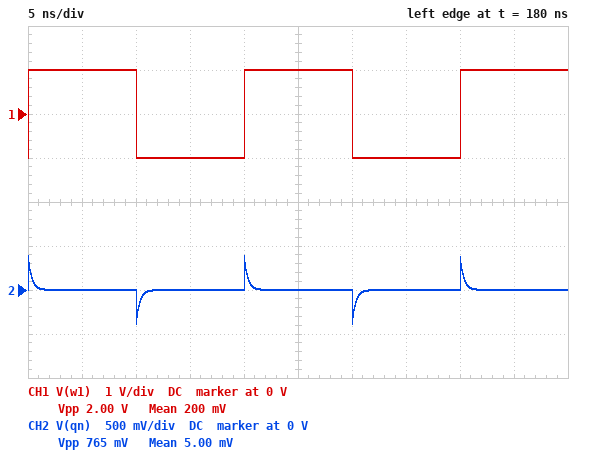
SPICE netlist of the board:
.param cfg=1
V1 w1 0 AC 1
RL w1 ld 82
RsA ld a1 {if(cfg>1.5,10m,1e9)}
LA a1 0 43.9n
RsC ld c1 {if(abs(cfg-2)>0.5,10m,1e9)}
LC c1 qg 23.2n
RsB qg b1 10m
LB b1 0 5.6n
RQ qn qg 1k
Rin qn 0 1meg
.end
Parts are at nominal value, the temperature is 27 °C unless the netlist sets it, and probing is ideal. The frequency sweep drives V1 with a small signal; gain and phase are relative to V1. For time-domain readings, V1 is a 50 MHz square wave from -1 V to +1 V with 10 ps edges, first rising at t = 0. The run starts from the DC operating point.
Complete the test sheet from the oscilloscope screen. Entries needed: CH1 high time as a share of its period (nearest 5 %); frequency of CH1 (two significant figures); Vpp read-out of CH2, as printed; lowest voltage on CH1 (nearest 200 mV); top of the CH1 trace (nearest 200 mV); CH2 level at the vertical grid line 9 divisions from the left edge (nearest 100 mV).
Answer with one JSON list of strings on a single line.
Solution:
["50 %", "50 MHz", "765 mV", "-1.0 V", "1.0 V", "0 V"]
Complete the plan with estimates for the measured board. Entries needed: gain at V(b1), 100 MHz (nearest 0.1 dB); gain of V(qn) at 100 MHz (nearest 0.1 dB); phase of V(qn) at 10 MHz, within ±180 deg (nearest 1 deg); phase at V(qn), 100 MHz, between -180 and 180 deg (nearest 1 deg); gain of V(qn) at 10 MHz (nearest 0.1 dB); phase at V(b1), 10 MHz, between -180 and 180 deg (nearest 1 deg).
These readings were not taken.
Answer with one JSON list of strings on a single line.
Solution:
["-27.6 dB", "-27.6 dB", "87 deg", "77 deg", "-47.4 dB", "89 deg"]
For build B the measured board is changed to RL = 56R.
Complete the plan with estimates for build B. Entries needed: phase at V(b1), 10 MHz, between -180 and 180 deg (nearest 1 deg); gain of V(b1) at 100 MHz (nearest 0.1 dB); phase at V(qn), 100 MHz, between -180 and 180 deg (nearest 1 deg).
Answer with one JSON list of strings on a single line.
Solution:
["88 deg", "-24.5 dB", "72 deg"]
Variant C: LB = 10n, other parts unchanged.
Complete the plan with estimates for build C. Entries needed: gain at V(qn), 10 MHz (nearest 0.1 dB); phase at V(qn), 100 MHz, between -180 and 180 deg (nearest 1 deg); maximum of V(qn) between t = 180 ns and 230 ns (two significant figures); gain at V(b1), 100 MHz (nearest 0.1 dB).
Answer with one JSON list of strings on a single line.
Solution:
["-42.3 dB", "76 deg", "590 mV", "-22.6 dB"]
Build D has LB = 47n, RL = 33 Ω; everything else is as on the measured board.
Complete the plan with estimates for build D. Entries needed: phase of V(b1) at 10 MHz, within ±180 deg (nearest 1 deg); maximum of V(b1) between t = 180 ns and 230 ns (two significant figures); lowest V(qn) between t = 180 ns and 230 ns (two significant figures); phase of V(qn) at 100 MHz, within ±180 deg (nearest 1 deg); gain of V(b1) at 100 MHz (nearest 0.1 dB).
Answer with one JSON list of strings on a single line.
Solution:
["82 deg", "1.3 V", "-1.3 V", "37 deg", "-5.4 dB"]
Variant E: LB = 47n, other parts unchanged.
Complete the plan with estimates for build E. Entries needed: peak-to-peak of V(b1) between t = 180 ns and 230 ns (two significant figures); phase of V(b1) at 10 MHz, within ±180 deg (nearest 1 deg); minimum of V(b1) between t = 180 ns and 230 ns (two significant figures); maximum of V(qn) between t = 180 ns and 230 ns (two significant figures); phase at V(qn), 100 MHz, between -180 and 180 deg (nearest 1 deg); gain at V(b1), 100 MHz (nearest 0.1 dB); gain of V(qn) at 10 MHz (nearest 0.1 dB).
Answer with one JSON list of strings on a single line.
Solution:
["2.7 V", "87 deg", "-1.3 V", "1.3 V", "62 deg", "-10.0 dB", "-28.9 dB"]
